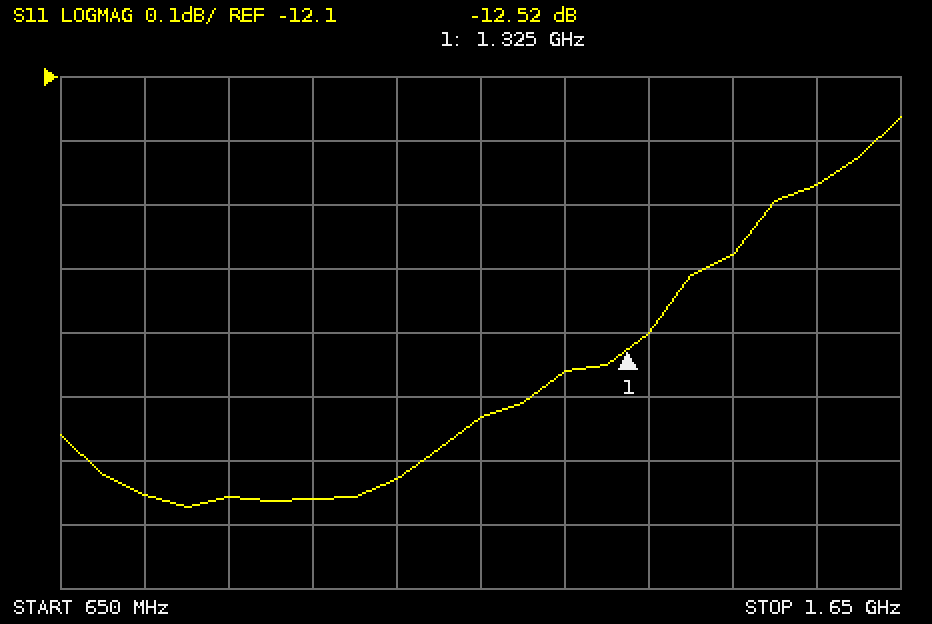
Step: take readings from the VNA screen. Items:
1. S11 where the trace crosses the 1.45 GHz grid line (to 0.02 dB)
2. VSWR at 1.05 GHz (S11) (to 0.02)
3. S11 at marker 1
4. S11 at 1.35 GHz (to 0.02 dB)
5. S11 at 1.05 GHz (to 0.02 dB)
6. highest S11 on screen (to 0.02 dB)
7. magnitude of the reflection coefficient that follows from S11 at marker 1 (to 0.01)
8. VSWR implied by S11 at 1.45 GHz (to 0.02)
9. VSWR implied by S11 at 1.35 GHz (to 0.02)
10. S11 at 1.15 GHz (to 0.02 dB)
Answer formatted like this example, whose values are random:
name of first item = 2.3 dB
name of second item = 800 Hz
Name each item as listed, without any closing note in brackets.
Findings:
S11 where the trace crosses the 1.45 GHz grid line = -12.38 dB
VSWR at 1.05 GHz (S11) = 1.60
S11 at marker 1 = -12.52 dB
S11 at 1.35 GHz = -12.50 dB
S11 at 1.05 GHz = -12.72 dB
highest S11 on screen = -12.16 dB
magnitude of the reflection coefficient that follows from S11 at marker 1 = 0.24
VSWR implied by S11 at 1.45 GHz = 1.64
VSWR implied by S11 at 1.35 GHz = 1.62
S11 at 1.15 GHz = -12.64 dB
